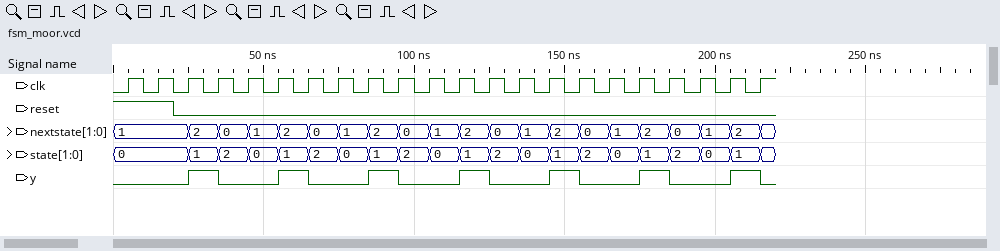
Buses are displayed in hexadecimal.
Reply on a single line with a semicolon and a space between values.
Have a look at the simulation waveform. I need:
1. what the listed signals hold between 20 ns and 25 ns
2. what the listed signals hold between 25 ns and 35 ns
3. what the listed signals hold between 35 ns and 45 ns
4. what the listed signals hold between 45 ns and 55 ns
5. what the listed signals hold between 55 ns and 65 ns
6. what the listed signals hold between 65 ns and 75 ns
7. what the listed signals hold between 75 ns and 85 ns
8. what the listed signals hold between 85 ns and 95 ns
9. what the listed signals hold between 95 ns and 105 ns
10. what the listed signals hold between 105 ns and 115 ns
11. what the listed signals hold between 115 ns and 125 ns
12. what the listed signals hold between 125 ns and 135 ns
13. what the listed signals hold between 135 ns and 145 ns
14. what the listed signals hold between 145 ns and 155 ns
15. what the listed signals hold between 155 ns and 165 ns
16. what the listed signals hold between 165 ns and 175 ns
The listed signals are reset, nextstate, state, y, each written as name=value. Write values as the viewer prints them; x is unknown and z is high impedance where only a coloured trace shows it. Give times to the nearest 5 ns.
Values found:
reset=0, nextstate=1, state=0, y=0; reset=0, nextstate=2, state=1, y=1; reset=0, nextstate=0, state=2, y=0; reset=0, nextstate=1, state=0, y=0; reset=0, nextstate=2, state=1, y=1; reset=0, nextstate=0, state=2, y=0; reset=0, nextstate=1, state=0, y=0; reset=0, nextstate=2, state=1, y=1; reset=0, nextstate=0, state=2, y=0; reset=0, nextstate=1, state=0, y=0; reset=0, nextstate=2, state=1, y=1; reset=0, nextstate=0, state=2, y=0; reset=0, nextstate=1, state=0, y=0; reset=0, nextstate=2, state=1, y=1; reset=0, nextstate=0, state=2, y=0; reset=0, nextstate=1, state=0, y=0
